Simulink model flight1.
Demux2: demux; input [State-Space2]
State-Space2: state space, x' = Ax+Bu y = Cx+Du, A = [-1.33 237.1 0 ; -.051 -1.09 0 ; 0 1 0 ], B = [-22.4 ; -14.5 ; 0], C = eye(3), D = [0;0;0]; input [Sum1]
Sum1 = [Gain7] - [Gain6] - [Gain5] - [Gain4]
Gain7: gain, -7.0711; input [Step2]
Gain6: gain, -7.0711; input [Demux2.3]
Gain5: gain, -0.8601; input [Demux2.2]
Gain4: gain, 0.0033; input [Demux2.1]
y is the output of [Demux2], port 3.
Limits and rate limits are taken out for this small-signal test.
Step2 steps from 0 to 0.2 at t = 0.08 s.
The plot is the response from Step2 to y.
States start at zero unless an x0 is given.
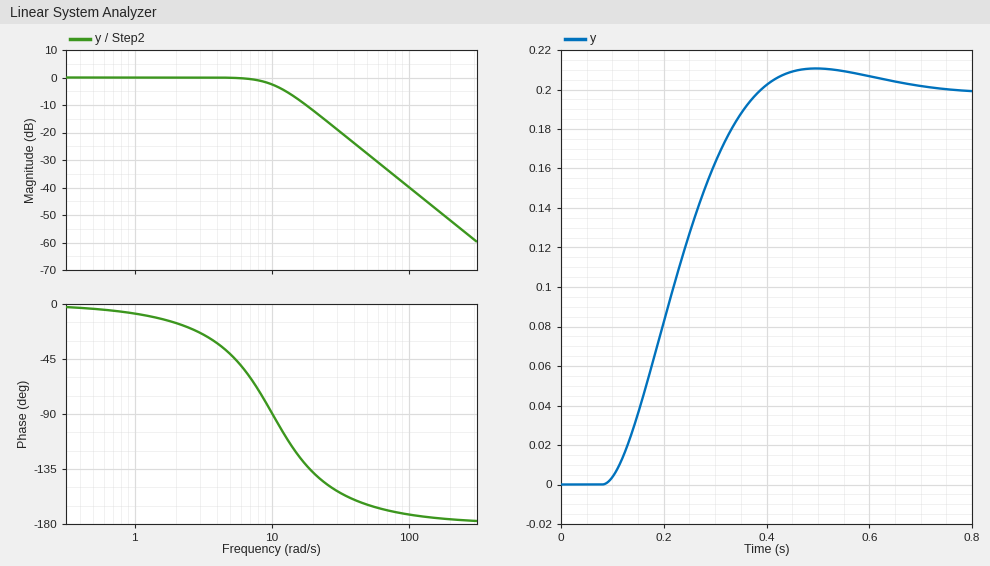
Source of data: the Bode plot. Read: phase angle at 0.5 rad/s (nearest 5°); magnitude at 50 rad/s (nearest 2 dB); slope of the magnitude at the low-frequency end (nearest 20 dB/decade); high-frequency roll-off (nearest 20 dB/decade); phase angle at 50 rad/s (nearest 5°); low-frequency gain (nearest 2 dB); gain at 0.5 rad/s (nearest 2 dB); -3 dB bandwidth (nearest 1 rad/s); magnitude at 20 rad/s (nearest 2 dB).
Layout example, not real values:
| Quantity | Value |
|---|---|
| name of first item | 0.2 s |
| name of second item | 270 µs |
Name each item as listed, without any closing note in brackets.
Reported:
| Quantity | Value |
|---|---|
| phase angle at 0.5 rad/s | -5° |
| magnitude at 50 rad/s | -28 dB |
| slope of the magnitude at the low-frequency end | 0 dB/decade |
| high-frequency roll-off | -40 dB/decade |
| phase angle at 50 rad/s | -165° |
| low-frequency gain | 0 dB |
| gain at 0.5 rad/s | 0 dB |
| -3 dB bandwidth | 11 rad/s |
| magnitude at 20 rad/s | -12 dB |
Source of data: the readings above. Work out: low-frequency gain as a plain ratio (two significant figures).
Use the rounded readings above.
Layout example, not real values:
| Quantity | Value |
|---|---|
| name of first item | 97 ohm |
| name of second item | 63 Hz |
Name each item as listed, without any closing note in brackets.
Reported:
| Quantity | Value |
|---|---|
| low-frequency gain as a plain ratio | 1.0 |
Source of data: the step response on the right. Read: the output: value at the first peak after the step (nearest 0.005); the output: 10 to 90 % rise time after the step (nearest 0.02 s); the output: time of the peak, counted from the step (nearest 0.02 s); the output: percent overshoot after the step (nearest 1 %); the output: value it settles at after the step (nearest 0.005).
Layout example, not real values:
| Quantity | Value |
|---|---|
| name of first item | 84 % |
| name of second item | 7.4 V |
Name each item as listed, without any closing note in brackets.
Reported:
| Quantity | Value |
|---|---|
| the output: value at the first peak after the step | 0.210 |
| the output: 10 to 90 % rise time after the step | 0.20 s |
| the output: time of the peak, counted from the step | 0.42 s |
| the output: percent overshoot after the step | 5 % |
| the output: value it settles at after the step | 0.200 |
